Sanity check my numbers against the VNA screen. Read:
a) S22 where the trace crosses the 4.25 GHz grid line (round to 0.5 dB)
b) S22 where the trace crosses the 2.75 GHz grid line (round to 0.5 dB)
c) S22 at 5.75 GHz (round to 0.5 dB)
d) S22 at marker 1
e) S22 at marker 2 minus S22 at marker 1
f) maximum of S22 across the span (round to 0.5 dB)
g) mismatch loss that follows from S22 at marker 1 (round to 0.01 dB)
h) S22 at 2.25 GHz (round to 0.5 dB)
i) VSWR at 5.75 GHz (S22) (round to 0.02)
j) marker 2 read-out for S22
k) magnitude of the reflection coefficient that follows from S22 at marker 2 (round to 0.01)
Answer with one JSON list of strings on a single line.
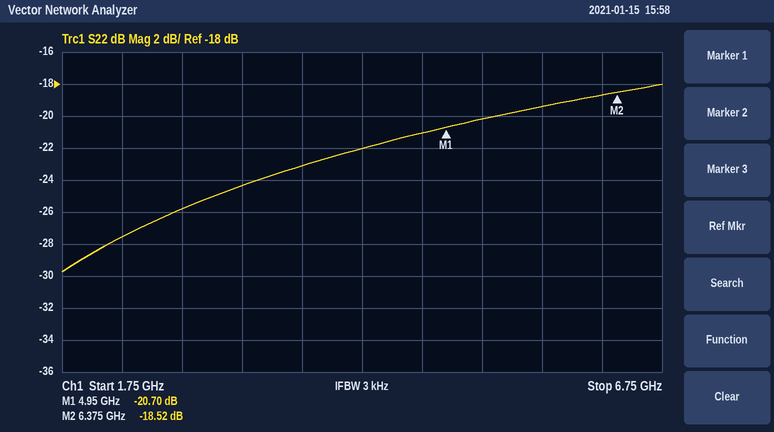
["-22.0 dB", "-26.0 dB", "-19.5 dB", "-20.70 dB", "2.18 dB", "-18.0 dB", "0.04 dB", "-27.5 dB", "1.24", "-18.52 dB", "0.12"]
